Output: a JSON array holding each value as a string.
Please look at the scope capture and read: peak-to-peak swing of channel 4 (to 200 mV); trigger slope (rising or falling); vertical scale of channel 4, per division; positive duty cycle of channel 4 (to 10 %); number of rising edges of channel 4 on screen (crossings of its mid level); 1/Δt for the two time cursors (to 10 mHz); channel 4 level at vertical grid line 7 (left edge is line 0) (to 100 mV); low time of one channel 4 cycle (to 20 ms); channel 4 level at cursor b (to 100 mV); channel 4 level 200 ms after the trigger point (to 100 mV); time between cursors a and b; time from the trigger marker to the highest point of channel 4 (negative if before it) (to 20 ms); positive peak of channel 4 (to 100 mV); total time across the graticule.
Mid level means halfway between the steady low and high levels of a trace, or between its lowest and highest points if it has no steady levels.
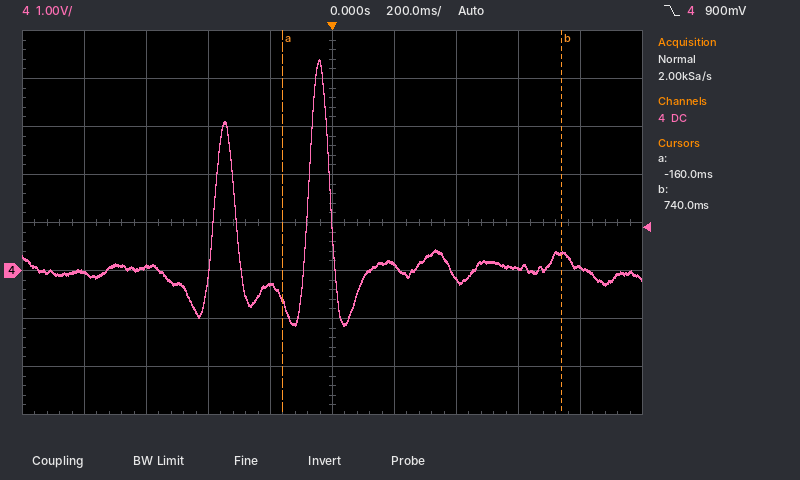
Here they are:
["5.6 V", "falling", "1 V", "20 %", "2", "1.11 Hz", "-200 mV", "240 ms", "400 mV", "100 mV", "900 ms", "-40 ms", "4.4 V", "2 s"]
